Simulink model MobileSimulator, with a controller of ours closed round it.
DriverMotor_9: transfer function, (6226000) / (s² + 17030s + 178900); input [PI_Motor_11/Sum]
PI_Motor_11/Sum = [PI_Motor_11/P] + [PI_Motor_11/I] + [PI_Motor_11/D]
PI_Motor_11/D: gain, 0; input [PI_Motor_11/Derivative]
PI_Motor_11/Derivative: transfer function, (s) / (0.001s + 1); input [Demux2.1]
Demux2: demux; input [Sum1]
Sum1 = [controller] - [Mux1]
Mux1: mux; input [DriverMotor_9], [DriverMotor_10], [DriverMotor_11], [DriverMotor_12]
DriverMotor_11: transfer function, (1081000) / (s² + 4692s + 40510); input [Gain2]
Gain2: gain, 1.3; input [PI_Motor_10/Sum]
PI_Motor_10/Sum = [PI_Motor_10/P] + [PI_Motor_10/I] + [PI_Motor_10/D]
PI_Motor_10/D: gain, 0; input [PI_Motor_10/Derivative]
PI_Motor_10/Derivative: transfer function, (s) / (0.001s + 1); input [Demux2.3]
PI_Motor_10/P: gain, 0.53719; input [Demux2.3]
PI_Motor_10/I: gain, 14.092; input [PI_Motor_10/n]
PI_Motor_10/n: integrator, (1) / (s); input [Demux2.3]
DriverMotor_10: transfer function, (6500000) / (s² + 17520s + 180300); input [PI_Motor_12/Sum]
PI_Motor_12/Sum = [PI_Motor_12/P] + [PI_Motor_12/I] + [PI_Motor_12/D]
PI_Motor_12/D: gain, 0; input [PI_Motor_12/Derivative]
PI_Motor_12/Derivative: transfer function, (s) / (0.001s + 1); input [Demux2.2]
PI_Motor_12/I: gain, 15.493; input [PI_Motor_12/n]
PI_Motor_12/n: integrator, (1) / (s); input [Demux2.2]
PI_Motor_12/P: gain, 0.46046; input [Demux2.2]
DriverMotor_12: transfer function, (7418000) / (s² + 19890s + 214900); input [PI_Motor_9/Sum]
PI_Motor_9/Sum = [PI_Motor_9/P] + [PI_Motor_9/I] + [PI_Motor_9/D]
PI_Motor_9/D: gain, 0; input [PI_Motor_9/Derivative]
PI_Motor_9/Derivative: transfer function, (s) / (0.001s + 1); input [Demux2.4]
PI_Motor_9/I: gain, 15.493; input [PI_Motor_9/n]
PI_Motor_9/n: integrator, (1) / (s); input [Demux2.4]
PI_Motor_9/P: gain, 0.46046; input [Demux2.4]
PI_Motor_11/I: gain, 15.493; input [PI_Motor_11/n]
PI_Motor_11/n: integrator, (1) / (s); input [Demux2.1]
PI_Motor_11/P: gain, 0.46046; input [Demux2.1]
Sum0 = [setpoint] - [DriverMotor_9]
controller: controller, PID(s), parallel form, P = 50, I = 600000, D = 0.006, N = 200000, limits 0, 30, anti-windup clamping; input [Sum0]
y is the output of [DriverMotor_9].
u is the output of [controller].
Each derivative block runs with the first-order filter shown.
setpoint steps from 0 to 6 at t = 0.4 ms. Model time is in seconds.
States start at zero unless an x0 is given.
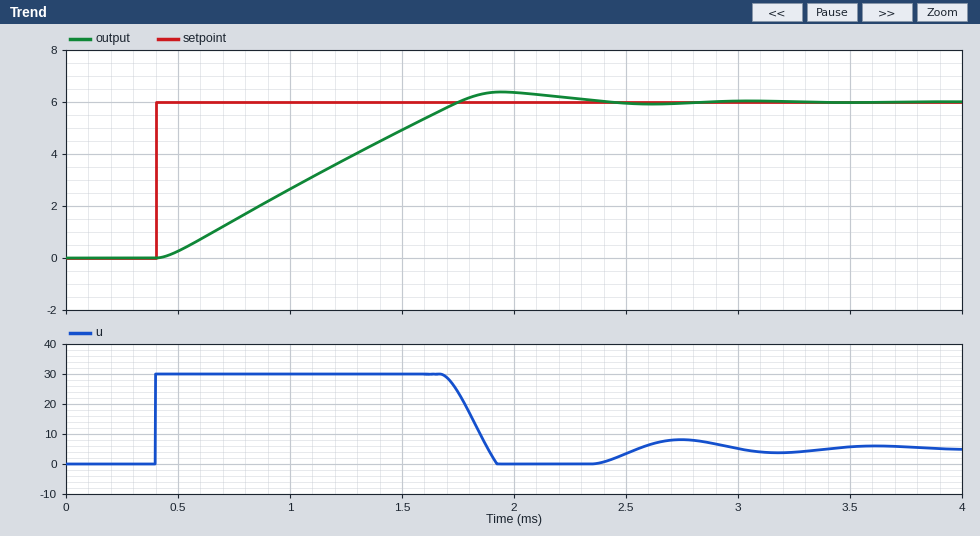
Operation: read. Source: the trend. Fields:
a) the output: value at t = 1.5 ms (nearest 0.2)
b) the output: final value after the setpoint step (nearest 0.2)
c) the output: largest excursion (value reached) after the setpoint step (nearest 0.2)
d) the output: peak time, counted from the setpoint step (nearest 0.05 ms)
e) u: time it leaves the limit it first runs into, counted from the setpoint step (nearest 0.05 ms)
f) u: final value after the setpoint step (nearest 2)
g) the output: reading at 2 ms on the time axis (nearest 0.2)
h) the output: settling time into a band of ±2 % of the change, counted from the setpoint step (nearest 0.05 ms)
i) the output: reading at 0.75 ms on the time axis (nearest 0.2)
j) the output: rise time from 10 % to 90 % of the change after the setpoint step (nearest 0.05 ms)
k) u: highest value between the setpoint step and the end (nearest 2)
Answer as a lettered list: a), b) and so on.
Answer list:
a) 5.0
b) 6.0
c) 6.4
d) 1.55 ms
e) 1.30 ms
f) 6
g) 6.4
h) 1.90 ms
i) 1.4
j) 1.05 ms
k) 30
